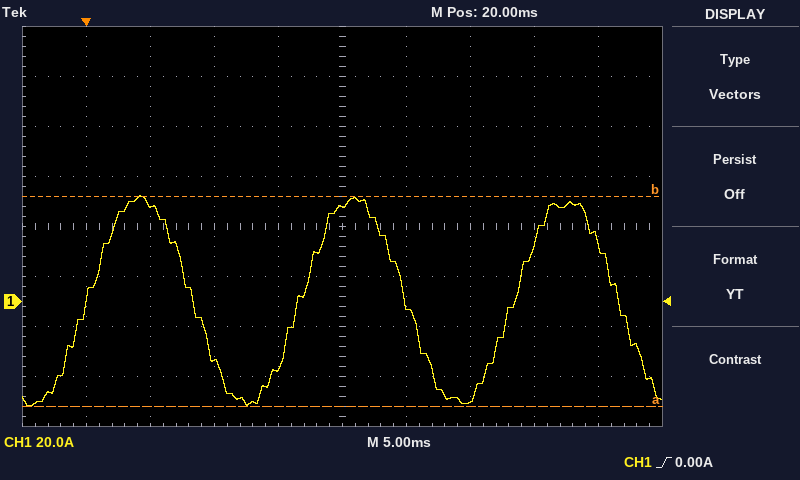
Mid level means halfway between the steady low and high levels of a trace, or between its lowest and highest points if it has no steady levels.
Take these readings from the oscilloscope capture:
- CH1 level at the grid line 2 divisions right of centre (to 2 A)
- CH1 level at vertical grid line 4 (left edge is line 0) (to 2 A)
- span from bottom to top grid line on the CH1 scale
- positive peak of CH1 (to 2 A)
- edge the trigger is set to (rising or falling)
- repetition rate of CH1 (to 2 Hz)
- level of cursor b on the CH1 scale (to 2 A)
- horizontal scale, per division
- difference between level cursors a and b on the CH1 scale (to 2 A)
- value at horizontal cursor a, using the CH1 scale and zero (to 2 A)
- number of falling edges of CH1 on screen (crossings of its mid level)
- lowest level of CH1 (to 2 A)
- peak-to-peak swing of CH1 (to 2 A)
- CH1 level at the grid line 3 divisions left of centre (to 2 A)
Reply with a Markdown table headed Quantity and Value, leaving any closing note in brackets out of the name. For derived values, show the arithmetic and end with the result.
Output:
| Quantity | Value |
|---|---|
| CH1 level at the grid line 2 divisions right of centre | -40 A |
| CH1 level at vertical grid line 4 (left edge is line 0) | -26 A |
| span from bottom to top grid line on the CH1 scale | 160 A |
| positive peak of CH1 | 42 A |
| edge the trigger is set to | rising |
| repetition rate of CH1 | 60 Hz |
| level of cursor b on the CH1 scale | 42 A |
| horizontal scale, per division | 5 ms |
| difference between level cursors a and b on the CH1 scale | 84 A |
| value at horizontal cursor a, using the CH1 scale and zero | -42 A |
| number of falling edges of CH1 on screen | 3 |
| lowest level of CH1 | -42 A |
| peak-to-peak swing of CH1 | 42 A − (-42 A) = 84 A |
| CH1 level at the grid line 3 divisions left of centre | 38 A |
